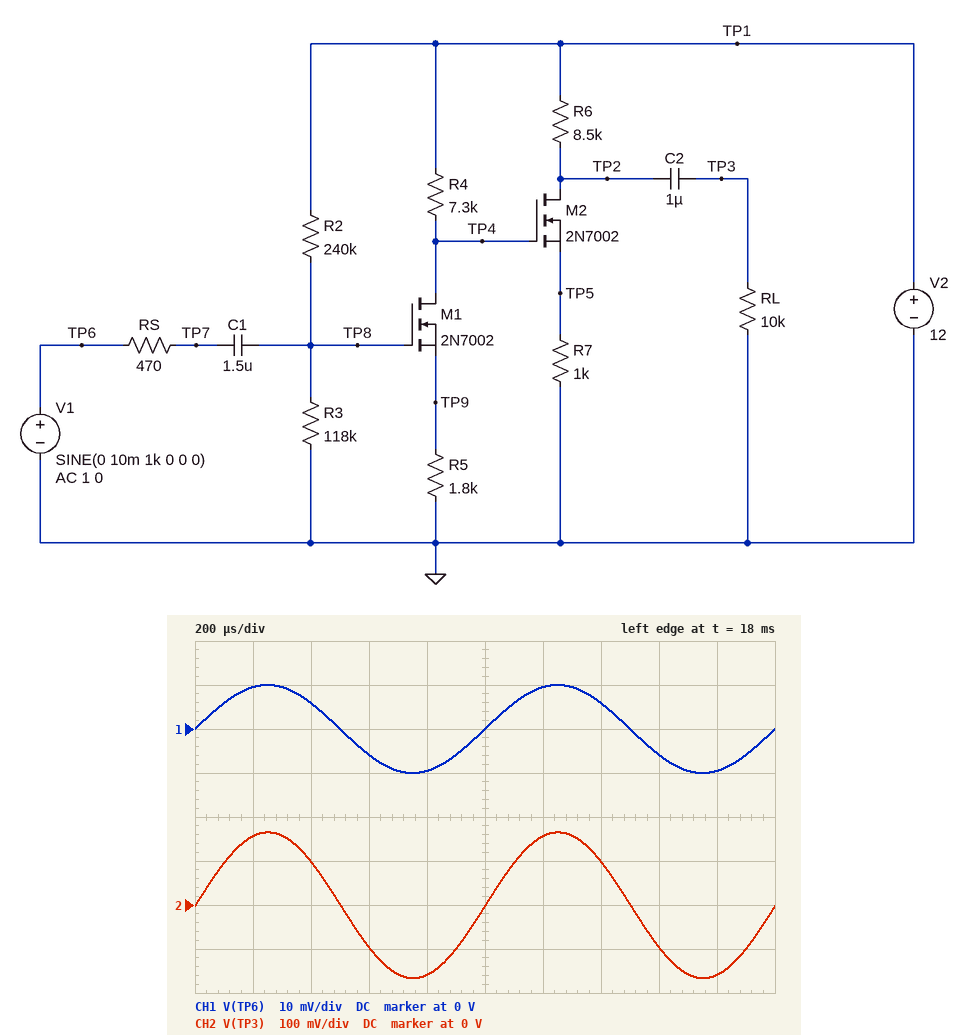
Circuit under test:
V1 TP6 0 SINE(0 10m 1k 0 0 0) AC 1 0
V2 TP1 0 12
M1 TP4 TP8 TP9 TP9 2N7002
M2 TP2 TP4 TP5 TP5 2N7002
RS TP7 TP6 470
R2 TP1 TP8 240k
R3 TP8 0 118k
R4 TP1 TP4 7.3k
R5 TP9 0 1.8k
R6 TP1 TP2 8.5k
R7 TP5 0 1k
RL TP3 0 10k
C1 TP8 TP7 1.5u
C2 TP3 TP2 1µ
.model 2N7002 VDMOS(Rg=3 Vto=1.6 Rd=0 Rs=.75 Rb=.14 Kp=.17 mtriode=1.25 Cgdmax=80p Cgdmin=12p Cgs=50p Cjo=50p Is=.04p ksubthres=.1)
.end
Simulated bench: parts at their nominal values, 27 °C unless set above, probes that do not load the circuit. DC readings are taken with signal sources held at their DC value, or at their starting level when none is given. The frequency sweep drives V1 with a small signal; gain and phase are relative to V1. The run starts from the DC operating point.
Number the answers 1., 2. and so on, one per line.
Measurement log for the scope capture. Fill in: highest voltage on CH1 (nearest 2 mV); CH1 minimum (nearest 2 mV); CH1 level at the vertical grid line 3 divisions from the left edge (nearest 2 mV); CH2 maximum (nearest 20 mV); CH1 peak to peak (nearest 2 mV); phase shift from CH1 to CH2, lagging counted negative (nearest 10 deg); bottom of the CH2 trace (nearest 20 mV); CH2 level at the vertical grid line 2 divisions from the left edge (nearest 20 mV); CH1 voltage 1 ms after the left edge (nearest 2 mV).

1. 10 mV
2. -10 mV
3. -6 mV
4. 160 mV
5. 20 mV
6. 0 deg
7. -160 mV
8. 100 mV
9. 0 V
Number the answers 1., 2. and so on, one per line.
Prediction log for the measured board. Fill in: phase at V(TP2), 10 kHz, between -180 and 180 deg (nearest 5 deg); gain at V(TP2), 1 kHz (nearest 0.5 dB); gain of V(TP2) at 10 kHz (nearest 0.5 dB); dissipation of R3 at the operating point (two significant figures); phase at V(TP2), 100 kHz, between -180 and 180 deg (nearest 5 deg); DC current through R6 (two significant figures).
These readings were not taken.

1. -15 deg
2. 24.5 dB
3. 24.0 dB
4. 130 µW
5. -75 deg
6. 1.1 mA
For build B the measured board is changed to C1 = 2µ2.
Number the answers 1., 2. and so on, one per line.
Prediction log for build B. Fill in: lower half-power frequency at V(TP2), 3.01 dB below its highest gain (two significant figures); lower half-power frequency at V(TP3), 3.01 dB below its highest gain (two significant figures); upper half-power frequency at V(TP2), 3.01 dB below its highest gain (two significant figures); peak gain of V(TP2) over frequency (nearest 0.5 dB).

1. 780 mHz
2. 8.7 Hz
3. 18 Hz
4. 29.0 dB
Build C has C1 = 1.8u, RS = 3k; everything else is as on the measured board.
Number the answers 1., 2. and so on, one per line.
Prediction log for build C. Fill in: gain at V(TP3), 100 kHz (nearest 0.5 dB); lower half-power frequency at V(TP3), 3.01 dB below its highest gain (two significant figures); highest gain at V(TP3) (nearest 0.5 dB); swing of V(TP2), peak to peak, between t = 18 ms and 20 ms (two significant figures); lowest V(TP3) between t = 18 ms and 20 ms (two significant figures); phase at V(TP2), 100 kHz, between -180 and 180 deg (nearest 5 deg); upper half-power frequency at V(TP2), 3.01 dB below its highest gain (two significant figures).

1. 15.0 dB
2. 8.7 Hz
3. 24.0 dB
4. 320 mV
5. -160 mV
6. -85 deg
7. 19 Hz
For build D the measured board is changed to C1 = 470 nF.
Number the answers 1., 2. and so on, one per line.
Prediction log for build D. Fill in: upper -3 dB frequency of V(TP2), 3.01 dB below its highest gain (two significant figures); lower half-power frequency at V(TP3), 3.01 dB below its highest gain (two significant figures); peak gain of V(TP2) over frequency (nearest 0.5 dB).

1. 16 kHz
2. 10 Hz
3. 27.0 dB
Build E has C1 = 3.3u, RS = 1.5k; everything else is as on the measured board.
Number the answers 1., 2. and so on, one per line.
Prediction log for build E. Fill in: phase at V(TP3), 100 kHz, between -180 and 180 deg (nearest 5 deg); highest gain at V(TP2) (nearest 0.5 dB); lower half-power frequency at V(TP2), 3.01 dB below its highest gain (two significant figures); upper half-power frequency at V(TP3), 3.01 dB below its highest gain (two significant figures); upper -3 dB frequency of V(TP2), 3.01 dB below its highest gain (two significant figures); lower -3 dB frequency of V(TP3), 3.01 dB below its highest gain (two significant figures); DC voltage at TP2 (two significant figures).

1. -80 deg
2. 29.0 dB
3. 540 mHz
4. 43 kHz
5. 16 Hz
6. 8.6 Hz
7. 2.4 V
